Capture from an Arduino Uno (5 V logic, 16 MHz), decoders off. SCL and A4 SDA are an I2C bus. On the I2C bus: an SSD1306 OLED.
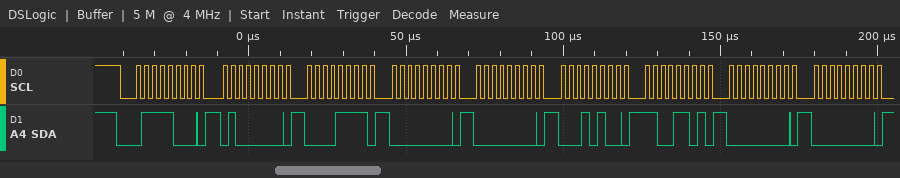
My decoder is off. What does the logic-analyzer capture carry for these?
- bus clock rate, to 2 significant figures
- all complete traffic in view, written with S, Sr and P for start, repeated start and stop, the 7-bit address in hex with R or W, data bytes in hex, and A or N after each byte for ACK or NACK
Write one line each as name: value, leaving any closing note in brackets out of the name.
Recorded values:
bus clock rate, to 2 significant figures: 400 kHz
all complete traffic in view, written with S, Sr and P for start, repeated start and stop, the 7-bit address in hex with R or W, data bytes in hex, and A or N after each byte for ACK or NACK: S 3CW A 40 A 0F A 00 A 00 A 14 A CD A 00 A 00 A
